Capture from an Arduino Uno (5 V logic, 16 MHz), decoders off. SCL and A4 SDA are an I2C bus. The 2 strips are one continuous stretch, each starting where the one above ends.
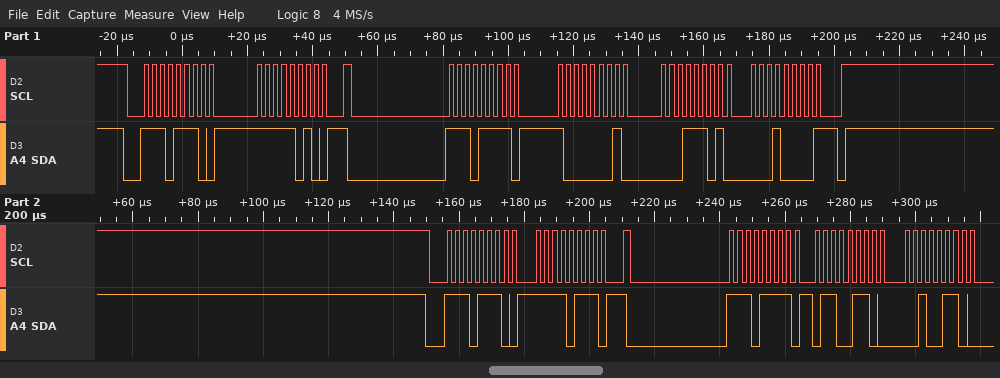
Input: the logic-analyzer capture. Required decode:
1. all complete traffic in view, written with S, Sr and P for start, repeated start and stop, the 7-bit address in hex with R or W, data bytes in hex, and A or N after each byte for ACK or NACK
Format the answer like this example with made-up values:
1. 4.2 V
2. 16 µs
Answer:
1. S 77W A FA A Sr 77R A 81 A 1D A 10 N P S 77W A F7 A Sr 77R A 66 A 26 A
